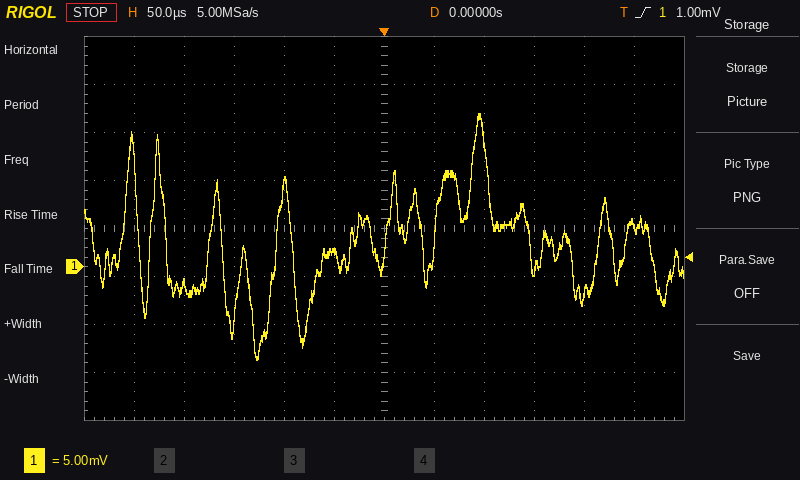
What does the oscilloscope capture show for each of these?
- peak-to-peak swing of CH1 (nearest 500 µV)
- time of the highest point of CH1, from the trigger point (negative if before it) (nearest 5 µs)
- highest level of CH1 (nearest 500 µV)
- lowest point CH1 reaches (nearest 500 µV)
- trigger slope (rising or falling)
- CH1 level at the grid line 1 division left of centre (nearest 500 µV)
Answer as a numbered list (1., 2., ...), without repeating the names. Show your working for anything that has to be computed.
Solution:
1. 16.0 mV − (-9.5 mV) = 25.5 mV
2. +95 µs
3. 16.0 mV
4. -9.5 mV
5. rising
6. 1.5 mV
